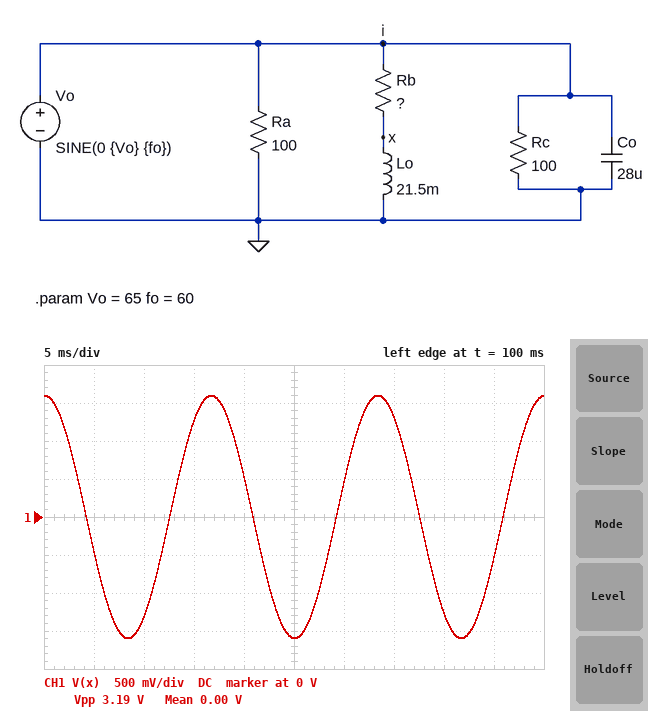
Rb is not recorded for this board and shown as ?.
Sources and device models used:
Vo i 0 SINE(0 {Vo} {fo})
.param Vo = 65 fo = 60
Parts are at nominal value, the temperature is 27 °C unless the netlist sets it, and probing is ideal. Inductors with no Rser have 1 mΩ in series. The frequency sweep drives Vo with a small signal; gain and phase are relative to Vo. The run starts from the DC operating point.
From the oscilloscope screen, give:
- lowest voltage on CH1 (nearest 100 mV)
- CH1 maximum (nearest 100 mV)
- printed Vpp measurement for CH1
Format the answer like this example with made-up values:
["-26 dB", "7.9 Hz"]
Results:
["-1.6 V", "1.6 V", "3.19 V"]
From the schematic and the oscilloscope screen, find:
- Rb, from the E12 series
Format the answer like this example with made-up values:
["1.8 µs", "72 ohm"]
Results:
["330 Ω"]
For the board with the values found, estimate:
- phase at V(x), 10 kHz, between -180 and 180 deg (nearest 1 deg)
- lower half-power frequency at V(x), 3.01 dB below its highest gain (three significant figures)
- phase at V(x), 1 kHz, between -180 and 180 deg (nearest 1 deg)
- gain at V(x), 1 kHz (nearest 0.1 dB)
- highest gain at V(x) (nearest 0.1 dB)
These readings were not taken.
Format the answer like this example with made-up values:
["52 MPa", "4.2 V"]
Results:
["14 deg", "2.44 kHz", "68 deg", "-8.4 dB", "0 dB"]
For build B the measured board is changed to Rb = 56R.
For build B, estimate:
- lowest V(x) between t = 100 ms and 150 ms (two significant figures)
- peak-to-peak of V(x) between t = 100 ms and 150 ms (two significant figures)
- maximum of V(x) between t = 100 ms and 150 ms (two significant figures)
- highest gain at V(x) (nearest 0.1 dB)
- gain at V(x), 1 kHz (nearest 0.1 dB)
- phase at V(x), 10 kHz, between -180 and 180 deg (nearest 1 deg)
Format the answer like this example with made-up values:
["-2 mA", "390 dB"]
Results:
["-9.3 V", "19 V", "9.3 V", "0 dB", "-0.7 dB", "2 deg"]
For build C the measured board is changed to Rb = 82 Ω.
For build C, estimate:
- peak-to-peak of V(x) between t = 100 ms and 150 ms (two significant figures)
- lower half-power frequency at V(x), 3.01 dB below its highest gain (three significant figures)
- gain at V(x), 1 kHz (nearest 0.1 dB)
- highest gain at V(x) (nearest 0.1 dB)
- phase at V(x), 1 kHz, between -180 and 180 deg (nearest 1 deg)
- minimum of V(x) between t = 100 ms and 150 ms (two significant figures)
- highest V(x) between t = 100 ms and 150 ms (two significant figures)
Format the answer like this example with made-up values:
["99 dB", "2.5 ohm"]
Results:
["13 V", "607 Hz", "-1.4 dB", "0 dB", "31 deg", "-6.4 V", "6.4 V"]
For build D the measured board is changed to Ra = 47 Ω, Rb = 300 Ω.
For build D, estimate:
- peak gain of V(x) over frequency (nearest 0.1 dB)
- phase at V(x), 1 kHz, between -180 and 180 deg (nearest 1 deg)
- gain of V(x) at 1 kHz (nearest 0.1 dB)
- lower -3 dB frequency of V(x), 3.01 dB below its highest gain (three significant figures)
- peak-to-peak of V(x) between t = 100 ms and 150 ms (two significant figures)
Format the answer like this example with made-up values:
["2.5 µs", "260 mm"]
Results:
["0 dB", "66 deg", "-7.7 dB", "2.22 kHz", "3.5 V"]
